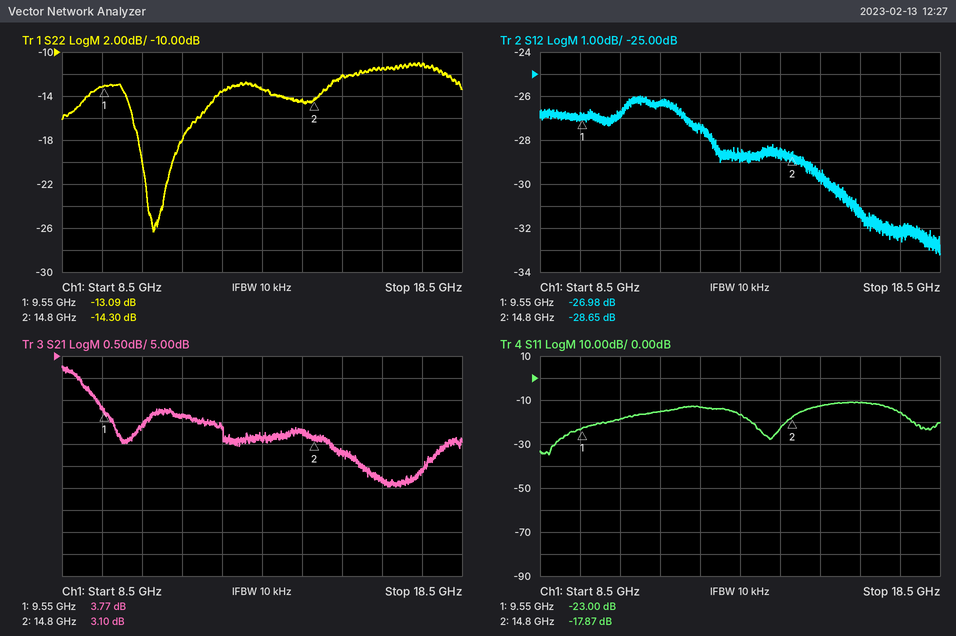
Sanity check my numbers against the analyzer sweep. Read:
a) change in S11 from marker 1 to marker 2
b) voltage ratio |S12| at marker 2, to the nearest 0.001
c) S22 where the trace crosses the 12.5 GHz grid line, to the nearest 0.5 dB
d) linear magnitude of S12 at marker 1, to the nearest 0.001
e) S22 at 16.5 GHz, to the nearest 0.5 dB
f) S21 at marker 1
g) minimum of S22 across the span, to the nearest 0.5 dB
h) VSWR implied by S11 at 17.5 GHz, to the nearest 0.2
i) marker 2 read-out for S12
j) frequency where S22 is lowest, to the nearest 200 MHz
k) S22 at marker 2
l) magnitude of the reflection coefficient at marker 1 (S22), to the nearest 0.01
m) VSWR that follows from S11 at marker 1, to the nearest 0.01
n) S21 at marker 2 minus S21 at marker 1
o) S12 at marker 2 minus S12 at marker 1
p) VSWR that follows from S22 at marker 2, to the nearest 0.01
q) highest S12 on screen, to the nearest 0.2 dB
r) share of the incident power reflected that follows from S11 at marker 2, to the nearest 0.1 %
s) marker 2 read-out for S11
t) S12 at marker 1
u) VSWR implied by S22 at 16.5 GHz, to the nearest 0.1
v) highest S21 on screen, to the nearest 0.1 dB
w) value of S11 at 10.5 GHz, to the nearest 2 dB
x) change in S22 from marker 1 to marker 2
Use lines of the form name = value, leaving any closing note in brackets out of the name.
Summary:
change in S11 from marker 1 to marker 2 = 5.13 dB
voltage ratio |S12| at marker 2, to the nearest 0.001 = 0.037
S22 where the trace crosses the 12.5 GHz grid line, to the nearest 0.5 dB = -13.5 dB
linear magnitude of S12 at marker 1, to the nearest 0.001 = 0.045
S22 at 16.5 GHz, to the nearest 0.5 dB = -11.5 dB
S21 at marker 1 = 3.77 dB
minimum of S22 across the span, to the nearest 0.5 dB = -26.5 dB
VSWR implied by S11 at 17.5 GHz, to the nearest 0.2 = 1.4
marker 2 read-out for S12 = -28.65 dB
frequency where S22 is lowest, to the nearest 200 MHz = 10.8 GHz
S22 at marker 2 = -14.30 dB
magnitude of the reflection coefficient at marker 1 (S22), to the nearest 0.01 = 0.22
VSWR that follows from S11 at marker 1, to the nearest 0.01 = 1.15
S21 at marker 2 minus S21 at marker 1 = -0.67 dB
S12 at marker 2 minus S12 at marker 1 = -1.67 dB
VSWR that follows from S22 at marker 2, to the nearest 0.01 = 1.48
highest S12 on screen, to the nearest 0.2 dB = -26.0 dB
share of the incident power reflected that follows from S11 at marker 2, to the nearest 0.1 % = 1.6 %
marker 2 read-out for S11 = -17.87 dB
S12 at marker 1 = -26.98 dB
VSWR implied by S22 at 16.5 GHz, to the nearest 0.1 = 1.7
highest S21 on screen, to the nearest 0.1 dB = 4.8 dB
value of S11 at 10.5 GHz, to the nearest 2 dB = -18 dB
change in S22 from marker 1 to marker 2 = -1.21 dB
